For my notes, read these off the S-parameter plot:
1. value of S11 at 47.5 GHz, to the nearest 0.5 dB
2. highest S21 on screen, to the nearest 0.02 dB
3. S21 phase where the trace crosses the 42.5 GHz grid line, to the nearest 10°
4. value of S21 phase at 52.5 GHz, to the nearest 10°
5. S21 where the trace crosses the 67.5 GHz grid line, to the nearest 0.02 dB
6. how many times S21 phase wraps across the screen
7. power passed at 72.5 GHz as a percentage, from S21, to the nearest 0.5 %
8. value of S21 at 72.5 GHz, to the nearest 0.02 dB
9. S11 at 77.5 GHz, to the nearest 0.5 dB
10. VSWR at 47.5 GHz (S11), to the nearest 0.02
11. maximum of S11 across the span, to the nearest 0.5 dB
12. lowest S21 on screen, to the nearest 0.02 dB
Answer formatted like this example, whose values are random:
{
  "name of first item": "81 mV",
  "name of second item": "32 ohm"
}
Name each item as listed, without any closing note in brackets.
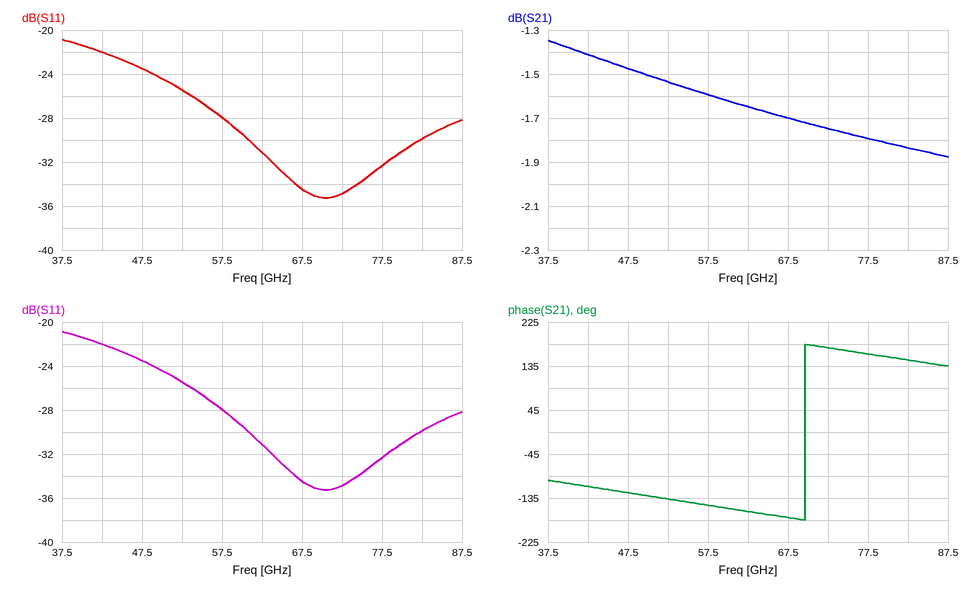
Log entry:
{
  "value of S11 at 47.5 GHz, to the nearest 0.5 dB": "-23.5 dB",
  "highest S21 on screen, to the nearest 0.02 dB": "-1.34 dB",
  "S21 phase where the trace crosses the 42.5 GHz grid line, to the nearest 10°": "-110°",
  "value of S21 phase at 52.5 GHz, to the nearest 10°": "-140°",
  "S21 where the trace crosses the 67.5 GHz grid line, to the nearest 0.02 dB": "-1.70 dB",
  "how many times S21 phase wraps across the screen": "1",
  "power passed at 72.5 GHz as a percentage, from S21, to the nearest 0.5 %": "67.0 %",
  "value of S21 at 72.5 GHz, to the nearest 0.02 dB": "-1.74 dB",
  "S11 at 77.5 GHz, to the nearest 0.5 dB": "-32.5 dB",
  "VSWR at 47.5 GHz (S11), to the nearest 0.02": "1.14",
  "maximum of S11 across the span, to the nearest 0.5 dB": "-21.0 dB",
  "lowest S21 on screen, to the nearest 0.02 dB": "-1.88 dB"
}
